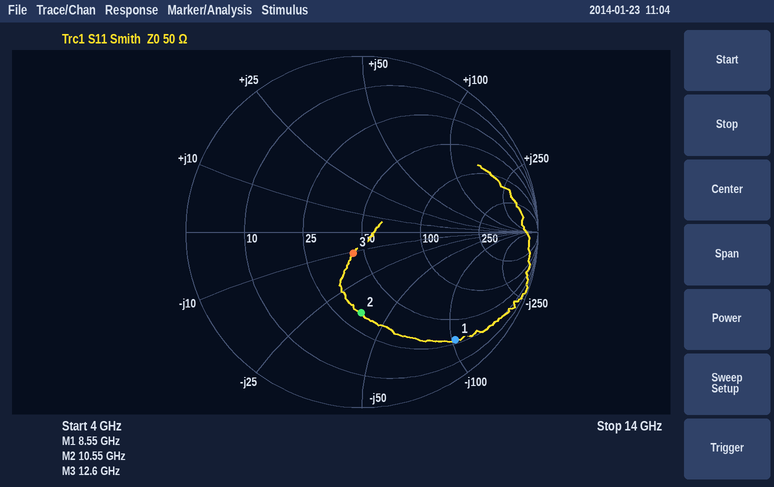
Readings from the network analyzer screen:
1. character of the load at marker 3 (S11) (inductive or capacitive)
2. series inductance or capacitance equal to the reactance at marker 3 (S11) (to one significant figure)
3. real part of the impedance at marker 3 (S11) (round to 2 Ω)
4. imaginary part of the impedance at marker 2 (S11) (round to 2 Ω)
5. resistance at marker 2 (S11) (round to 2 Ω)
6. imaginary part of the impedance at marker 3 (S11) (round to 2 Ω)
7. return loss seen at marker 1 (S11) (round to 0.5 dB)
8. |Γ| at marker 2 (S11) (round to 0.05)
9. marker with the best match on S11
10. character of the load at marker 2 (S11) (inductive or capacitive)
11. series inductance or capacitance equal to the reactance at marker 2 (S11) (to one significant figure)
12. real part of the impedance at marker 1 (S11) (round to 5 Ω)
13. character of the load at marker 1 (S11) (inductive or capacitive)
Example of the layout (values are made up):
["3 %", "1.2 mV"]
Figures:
["capacitive", "1 pF", "44 Ω", "-38 Ω", "32 Ω", "-10 Ω", "2.0 dB", "0.45", "marker 3", "capacitive", "400 fF", "30 Ω", "capacitive"]
